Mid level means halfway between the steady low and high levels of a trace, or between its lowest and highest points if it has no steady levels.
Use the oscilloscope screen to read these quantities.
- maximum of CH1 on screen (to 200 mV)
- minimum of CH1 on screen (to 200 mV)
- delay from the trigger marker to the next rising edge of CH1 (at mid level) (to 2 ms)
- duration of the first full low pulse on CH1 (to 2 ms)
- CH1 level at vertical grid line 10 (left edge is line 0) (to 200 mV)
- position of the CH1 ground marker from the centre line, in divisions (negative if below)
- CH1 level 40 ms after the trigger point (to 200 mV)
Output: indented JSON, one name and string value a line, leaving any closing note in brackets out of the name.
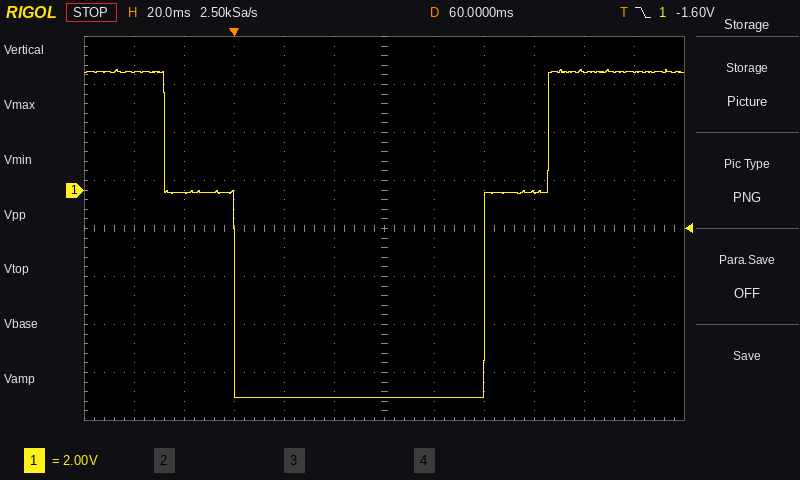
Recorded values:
{
  "maximum of CH1 on screen": "5.0 V",
  "minimum of CH1 on screen": "-8.6 V",
  "delay from the trigger marker to the next rising edge of CH1 (at mid level)": "100 ms",
  "duration of the first full low pulse on CH1": "100 ms",
  "CH1 level at vertical grid line 10 (left edge is line 0)": "5.0 V",
  "position of the CH1 ground marker from the centre line, in divisions": "+0.8 div",
  "CH1 level 40 ms after the trigger point": "-8.6 V"
}
